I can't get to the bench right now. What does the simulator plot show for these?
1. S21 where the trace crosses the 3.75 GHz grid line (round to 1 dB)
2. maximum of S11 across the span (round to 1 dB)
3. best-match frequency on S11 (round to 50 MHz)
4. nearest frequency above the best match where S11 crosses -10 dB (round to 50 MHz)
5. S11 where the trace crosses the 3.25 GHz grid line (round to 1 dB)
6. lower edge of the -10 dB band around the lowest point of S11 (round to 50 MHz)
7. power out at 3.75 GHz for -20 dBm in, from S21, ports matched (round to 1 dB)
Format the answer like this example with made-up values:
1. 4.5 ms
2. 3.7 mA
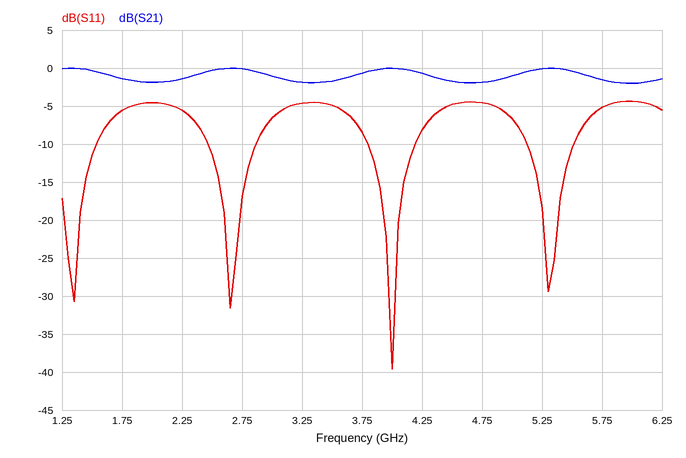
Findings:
1. -1 dB
2. -4 dB
3. 4.00 GHz
4. 4.20 GHz
5. -5 dB
6. 3.80 GHz
7. -21 dBm
